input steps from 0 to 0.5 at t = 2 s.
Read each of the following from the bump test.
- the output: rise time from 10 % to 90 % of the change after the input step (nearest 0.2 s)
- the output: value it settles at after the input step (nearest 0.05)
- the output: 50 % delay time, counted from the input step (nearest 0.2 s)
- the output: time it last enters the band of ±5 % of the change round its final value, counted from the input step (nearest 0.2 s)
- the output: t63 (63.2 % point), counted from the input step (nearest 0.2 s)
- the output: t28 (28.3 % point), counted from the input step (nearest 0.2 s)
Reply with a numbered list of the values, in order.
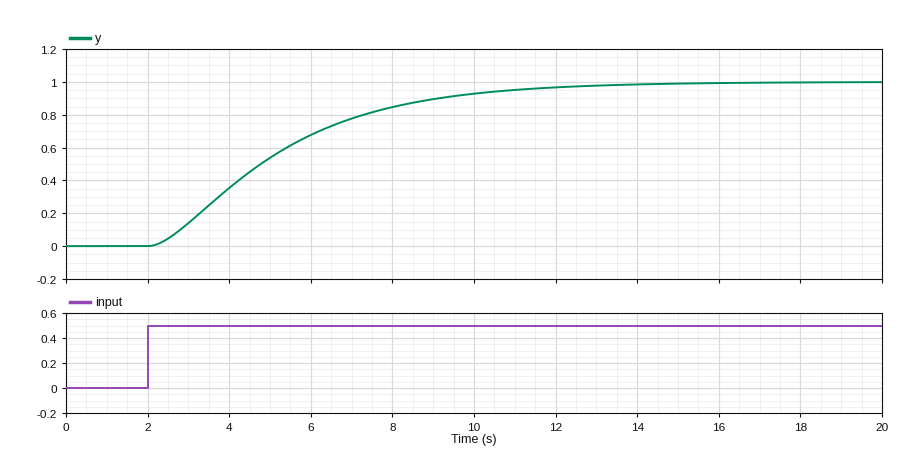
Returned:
1. 6.4 s
2. 1.00
3. 2.8 s
4. 9.0 s
5. 3.6 s
6. 1.6 s
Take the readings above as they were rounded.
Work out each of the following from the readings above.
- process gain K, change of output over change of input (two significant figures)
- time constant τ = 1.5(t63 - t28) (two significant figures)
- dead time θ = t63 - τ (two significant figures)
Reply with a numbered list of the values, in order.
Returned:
1. 2.0
2. 3.0 s
3. 0.60 s
